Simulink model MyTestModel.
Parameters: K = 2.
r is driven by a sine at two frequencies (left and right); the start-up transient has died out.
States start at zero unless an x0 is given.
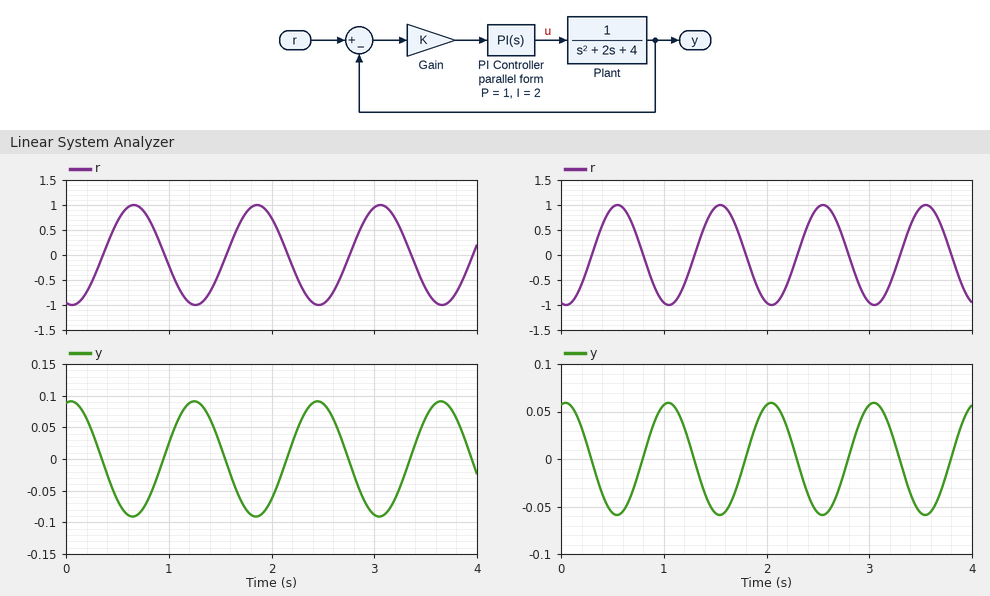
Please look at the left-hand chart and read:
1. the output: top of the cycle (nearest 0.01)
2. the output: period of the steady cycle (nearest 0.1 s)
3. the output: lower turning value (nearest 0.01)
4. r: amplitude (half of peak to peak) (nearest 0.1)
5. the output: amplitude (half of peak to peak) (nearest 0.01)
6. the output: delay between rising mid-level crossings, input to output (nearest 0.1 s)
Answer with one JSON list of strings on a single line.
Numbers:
["0.09", "1.2 s", "-0.09", "1.0", "0.09", "0.6 s"]
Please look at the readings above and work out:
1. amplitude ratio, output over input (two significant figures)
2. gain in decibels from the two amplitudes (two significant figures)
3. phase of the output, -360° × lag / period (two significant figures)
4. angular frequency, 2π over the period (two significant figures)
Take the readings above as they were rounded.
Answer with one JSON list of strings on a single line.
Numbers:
["0.090", "-21 dB", "-180°", "5.2 rad/s"]
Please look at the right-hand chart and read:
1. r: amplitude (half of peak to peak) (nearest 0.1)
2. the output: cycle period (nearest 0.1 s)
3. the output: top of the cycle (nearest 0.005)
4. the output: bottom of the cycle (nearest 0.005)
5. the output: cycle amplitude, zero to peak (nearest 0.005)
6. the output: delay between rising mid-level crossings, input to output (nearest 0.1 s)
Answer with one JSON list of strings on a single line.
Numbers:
["1.0", "1.0 s", "0.060", "-0.060", "0.060", "0.5 s"]
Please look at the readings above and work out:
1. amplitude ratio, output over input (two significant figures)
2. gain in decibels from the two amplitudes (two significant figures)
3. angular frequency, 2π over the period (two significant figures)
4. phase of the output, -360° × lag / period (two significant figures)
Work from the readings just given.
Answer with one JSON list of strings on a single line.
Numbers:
["0.060", "-24 dB", "6.3 rad/s", "-180°"]
